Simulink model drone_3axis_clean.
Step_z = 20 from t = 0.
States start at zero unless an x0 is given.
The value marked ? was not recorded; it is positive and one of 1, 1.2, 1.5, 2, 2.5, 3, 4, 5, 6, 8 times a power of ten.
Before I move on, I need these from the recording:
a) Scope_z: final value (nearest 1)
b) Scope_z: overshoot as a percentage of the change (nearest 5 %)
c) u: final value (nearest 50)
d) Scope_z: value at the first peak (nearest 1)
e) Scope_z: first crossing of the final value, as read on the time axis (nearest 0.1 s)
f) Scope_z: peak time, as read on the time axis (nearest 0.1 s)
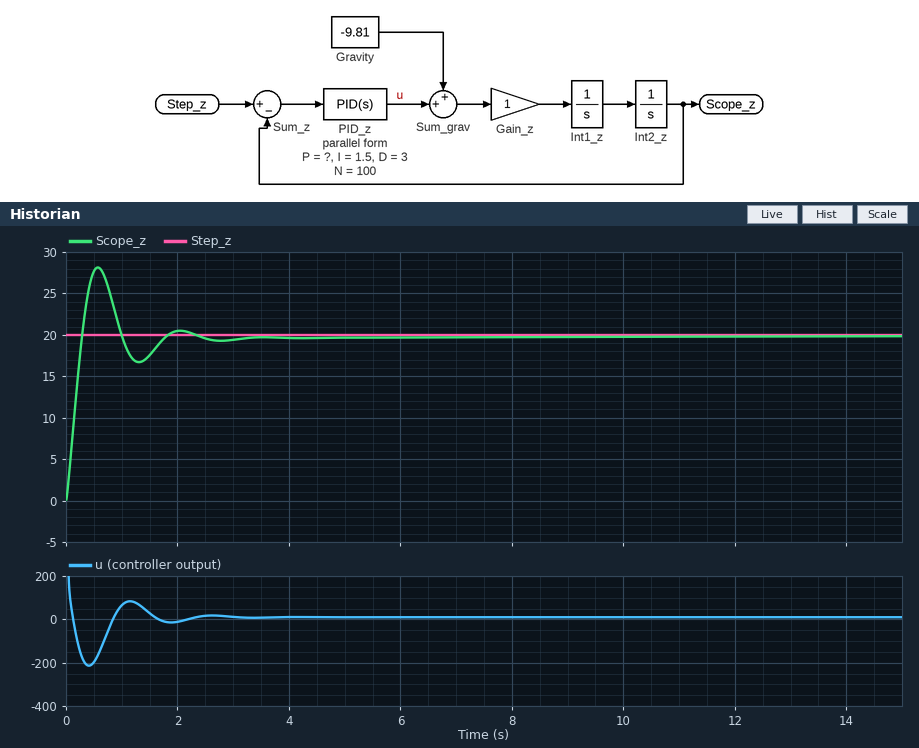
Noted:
20
40 %
0
28
0.3 s
0.6 s
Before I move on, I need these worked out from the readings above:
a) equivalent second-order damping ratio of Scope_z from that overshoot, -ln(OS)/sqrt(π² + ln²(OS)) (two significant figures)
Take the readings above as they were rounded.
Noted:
0.28
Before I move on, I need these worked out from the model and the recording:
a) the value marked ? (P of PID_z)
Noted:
20
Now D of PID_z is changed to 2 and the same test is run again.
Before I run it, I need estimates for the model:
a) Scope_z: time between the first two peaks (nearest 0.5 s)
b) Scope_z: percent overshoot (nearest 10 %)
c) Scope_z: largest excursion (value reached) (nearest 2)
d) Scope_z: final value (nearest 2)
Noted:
1.5 s
50 %
30
20
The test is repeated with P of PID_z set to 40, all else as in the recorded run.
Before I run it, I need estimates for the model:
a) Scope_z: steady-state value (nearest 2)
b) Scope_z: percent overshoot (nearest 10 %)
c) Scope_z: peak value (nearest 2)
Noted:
20
50 %
30
